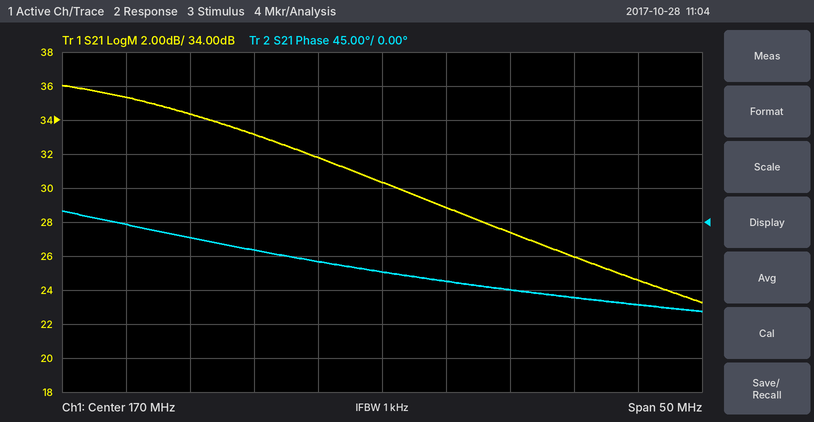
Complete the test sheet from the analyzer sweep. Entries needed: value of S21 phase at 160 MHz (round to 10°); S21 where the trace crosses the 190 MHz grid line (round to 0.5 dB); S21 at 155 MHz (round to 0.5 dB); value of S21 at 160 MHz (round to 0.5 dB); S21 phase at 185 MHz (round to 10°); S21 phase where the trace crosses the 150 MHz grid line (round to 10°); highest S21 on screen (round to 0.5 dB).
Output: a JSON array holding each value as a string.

["-40°", "24.5 dB", "34.5 dB", "33.0 dB", "-100°", "0°", "36.0 dB"]
